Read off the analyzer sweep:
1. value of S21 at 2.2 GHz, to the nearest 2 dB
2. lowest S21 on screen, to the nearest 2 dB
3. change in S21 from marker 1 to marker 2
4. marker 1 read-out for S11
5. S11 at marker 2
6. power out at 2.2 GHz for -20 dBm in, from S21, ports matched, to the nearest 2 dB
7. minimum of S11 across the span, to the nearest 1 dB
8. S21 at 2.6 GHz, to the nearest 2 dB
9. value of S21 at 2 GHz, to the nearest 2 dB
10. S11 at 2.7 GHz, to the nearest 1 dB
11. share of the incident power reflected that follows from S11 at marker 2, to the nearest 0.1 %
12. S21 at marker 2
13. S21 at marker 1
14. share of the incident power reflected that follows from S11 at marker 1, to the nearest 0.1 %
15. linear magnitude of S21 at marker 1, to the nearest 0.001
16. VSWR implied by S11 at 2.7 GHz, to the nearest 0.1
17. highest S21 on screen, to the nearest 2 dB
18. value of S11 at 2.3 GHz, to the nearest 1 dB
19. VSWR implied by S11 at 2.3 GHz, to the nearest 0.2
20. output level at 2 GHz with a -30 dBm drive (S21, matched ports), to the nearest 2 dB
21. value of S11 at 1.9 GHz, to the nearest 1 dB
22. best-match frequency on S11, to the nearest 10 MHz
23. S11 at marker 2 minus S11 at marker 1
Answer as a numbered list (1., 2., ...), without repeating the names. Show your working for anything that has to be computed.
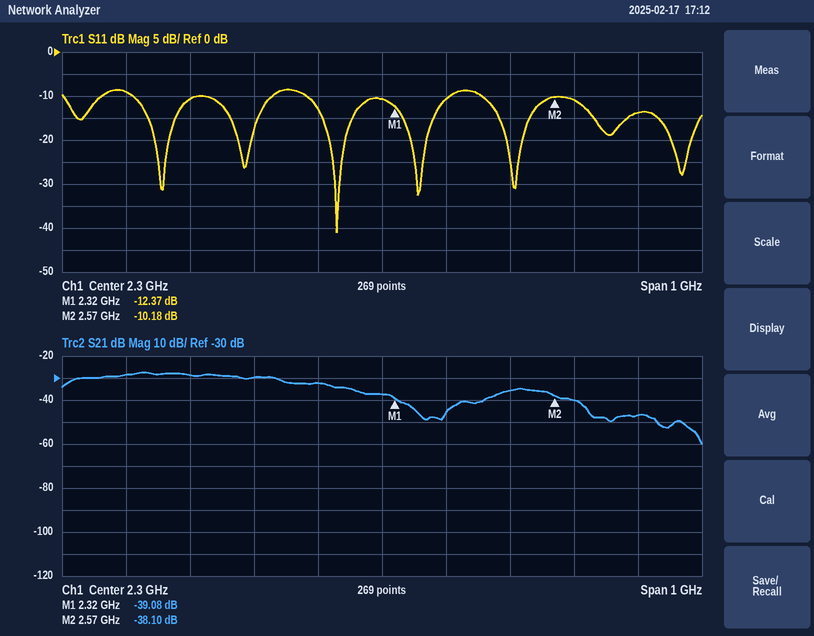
1. -32 dB
2. -60 dB
3. -38.1 − (-39.08) = 0.98 dB
4. -12.37 dB
5. -10.18 dB
6. -20 dBm + (-32 dB) = -52 dBm
7. -41 dB
8. -40 dB
9. -28 dB
10. -14 dB
11. 10^(-10.18/10) ≈ 9.6 %
12. -38.10 dB
13. -39.08 dB
14. 10^(-12.37/10) ≈ 5.8 %
15. 10^(-39.08/20) ≈ 0.011
16. |Γ| = 10^(-14/20) = 0.1995; VSWR = (1 + 0.1995)/(1 − 0.1995) ≈ 1.5
17. -28 dB
18. -11 dB
19. |Γ| = 10^(-11/20) = 0.2818; VSWR = (1 + 0.2818)/(1 − 0.2818) ≈ 1.8
20. -30 dBm + (-28 dB) = -58 dBm
21. -9 dB
22. 2.23 GHz
23. -10.18 − (-12.37) = 2.19 dB
